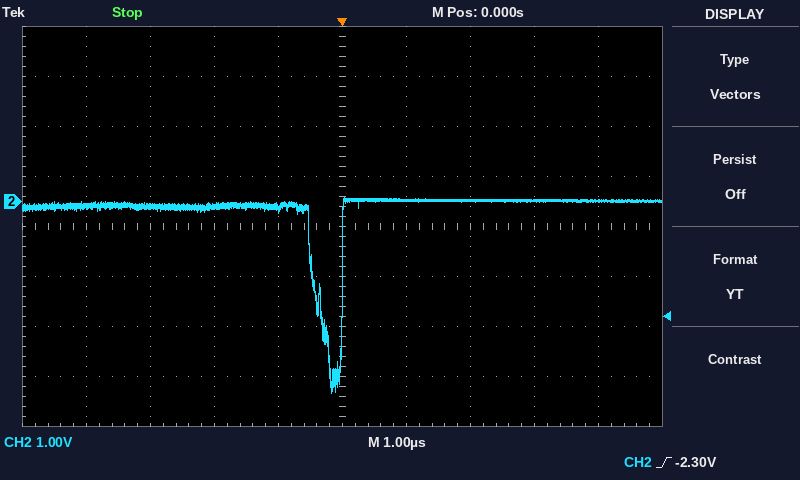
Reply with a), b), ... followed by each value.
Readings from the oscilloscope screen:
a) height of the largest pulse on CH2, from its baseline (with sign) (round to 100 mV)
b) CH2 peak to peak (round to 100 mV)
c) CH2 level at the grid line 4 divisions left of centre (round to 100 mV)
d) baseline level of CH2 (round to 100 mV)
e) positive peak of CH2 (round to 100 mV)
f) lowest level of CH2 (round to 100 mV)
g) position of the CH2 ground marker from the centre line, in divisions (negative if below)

a) -3.8 V
b) 3.9 V
c) -100 mV
d) 0.0 V
e) 100 mV
f) -3.8 V
g) +0.5 div
